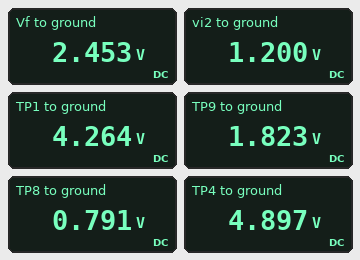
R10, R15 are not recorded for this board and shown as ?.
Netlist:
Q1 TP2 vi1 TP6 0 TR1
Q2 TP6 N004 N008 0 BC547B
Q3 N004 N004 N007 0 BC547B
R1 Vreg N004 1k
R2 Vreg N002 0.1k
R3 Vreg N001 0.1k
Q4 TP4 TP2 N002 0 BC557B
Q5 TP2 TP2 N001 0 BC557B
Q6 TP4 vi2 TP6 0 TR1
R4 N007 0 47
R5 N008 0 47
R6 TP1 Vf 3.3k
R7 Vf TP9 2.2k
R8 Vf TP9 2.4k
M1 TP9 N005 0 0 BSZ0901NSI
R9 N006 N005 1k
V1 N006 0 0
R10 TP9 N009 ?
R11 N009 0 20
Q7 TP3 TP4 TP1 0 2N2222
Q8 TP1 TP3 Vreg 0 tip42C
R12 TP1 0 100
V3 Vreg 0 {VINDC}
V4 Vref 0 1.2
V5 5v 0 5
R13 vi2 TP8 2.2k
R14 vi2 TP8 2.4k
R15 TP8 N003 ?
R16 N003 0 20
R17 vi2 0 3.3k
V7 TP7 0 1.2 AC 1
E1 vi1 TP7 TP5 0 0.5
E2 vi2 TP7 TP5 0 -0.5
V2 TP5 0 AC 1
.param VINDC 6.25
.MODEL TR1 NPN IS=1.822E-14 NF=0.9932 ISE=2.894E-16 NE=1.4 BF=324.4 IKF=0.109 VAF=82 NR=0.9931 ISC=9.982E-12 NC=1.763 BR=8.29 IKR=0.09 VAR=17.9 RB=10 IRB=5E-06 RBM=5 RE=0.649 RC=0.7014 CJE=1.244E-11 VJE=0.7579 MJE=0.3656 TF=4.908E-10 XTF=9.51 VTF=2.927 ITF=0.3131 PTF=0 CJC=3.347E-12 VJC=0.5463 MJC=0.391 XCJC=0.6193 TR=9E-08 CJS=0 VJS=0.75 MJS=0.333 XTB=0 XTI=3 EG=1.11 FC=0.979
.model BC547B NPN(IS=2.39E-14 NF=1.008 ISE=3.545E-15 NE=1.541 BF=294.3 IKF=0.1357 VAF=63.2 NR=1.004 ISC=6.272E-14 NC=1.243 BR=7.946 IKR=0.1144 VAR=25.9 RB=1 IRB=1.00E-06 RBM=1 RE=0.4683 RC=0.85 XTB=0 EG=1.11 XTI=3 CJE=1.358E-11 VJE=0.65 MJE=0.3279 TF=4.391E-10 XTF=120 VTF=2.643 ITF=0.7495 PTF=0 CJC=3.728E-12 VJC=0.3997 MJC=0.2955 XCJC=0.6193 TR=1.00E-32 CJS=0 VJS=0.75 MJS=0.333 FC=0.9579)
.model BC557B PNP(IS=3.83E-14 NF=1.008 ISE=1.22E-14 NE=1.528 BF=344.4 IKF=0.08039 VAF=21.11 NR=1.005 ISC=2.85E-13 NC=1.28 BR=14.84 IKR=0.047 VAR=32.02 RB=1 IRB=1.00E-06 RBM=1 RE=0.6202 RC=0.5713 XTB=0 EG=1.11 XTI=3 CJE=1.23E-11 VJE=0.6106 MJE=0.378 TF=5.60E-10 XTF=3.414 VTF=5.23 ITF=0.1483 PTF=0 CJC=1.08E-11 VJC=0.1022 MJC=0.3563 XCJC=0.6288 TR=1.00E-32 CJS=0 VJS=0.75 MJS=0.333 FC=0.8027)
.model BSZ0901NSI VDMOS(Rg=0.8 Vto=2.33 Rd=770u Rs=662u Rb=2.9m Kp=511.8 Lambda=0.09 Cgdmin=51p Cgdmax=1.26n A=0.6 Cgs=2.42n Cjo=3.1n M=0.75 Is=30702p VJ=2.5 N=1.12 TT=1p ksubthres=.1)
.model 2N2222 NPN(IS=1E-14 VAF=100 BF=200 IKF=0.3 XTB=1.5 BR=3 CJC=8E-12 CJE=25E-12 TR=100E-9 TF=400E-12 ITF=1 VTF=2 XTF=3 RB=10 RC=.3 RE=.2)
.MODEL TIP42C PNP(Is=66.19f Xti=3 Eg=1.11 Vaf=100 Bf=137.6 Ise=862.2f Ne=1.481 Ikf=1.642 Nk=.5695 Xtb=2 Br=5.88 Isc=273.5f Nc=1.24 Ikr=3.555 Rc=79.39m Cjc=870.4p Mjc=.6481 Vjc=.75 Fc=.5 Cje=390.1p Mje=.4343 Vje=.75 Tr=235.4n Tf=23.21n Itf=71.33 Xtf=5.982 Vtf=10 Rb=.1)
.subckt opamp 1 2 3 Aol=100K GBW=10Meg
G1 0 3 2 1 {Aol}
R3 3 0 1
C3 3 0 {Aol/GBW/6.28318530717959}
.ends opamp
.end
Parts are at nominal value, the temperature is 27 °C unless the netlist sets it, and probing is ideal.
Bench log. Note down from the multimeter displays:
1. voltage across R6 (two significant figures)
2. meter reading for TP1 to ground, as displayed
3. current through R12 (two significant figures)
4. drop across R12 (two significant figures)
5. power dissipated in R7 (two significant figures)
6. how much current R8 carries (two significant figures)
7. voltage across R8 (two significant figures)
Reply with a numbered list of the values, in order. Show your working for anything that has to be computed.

1. 4.264 V - 2.453 V = 1.8 V
2. 4.264 V
3. (4.264 V) / 100 Ω = 43 mA
4. 4.264 V = 4.3 V
5. (2.453 V - 1.823 V)^2 / 2.2 kΩ = 180 µW
6. (2.453 V - 1.823 V) / 2.4 kΩ = 260 µA
7. 2.453 V - 1.823 V = 630 mV
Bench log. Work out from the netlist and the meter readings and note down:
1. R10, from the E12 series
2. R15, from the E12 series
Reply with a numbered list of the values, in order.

1. 3.3 kΩ
2. 2.2 kΩ
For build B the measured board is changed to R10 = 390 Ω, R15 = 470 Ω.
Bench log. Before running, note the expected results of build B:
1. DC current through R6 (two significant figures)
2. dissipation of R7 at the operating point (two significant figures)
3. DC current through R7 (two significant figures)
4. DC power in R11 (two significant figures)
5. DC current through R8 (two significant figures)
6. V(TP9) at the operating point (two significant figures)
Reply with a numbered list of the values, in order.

1. 880 µA
2. 460 µW
3. 460 µA
4. 15 µW
5. 420 µA
6. 360 mV
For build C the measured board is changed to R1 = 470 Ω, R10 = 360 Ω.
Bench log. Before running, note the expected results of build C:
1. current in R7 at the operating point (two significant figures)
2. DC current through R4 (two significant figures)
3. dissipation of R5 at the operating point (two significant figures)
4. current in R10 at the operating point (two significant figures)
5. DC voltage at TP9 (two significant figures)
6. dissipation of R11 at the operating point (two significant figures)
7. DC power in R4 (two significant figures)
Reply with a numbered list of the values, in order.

1. 430 µA
2. 10 mA
3. 4.7 mW
4. 830 µA
5. 310 mV
6. 14 µW
7. 4.9 mW
